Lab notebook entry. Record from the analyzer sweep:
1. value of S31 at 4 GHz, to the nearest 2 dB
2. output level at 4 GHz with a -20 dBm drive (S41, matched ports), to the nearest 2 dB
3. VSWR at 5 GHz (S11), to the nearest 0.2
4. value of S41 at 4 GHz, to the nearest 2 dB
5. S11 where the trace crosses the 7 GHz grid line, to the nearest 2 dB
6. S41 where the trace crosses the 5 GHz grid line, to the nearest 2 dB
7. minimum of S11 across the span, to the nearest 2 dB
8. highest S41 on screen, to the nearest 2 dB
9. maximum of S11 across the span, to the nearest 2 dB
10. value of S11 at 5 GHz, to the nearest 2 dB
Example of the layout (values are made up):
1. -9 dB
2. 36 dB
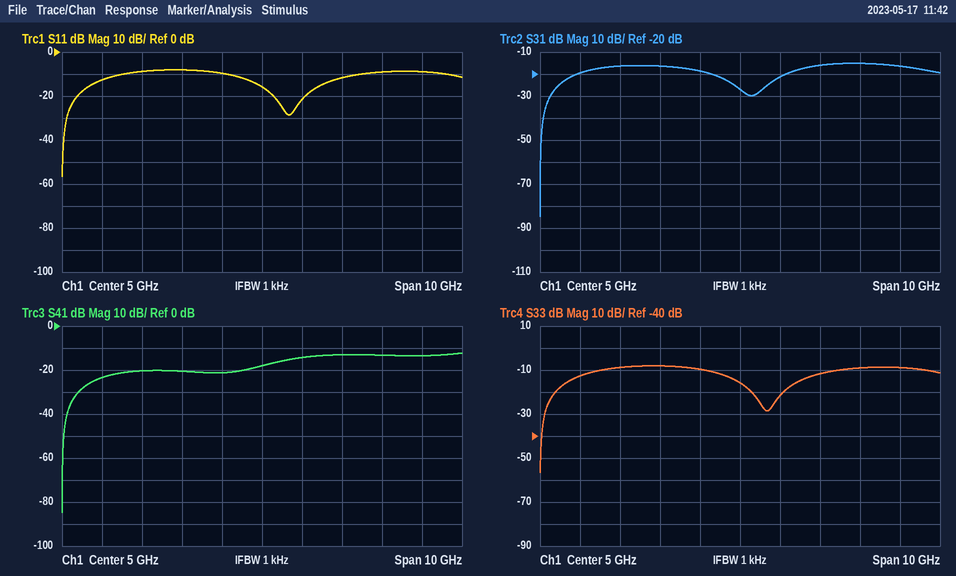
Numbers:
1. -18 dB
2. -42 dBm
3. 1.4
4. -22 dB
5. -12 dB
6. -18 dB
7. -56 dB
8. -12 dB
9. -8 dB
10. -16 dB
